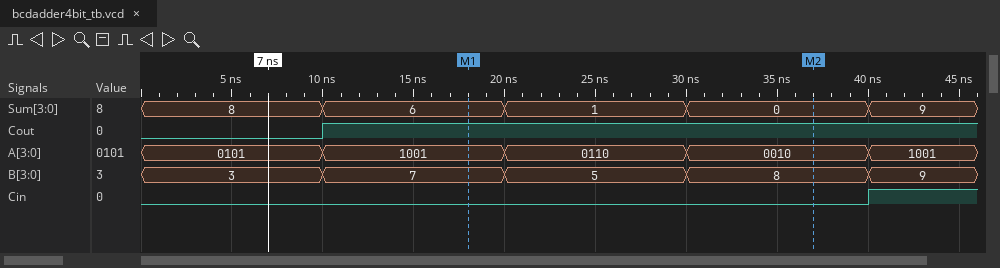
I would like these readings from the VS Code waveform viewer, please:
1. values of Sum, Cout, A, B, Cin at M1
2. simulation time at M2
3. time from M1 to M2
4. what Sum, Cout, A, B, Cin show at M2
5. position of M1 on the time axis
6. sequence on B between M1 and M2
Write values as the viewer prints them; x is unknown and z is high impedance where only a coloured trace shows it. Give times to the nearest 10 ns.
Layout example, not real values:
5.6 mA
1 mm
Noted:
Sum=6, Cout=1, A=1001, B=7, Cin=0
40 ns
20 ns
Sum=0, Cout=1, A=0010, B=8, Cin=0
20 ns
7, 5, 8
